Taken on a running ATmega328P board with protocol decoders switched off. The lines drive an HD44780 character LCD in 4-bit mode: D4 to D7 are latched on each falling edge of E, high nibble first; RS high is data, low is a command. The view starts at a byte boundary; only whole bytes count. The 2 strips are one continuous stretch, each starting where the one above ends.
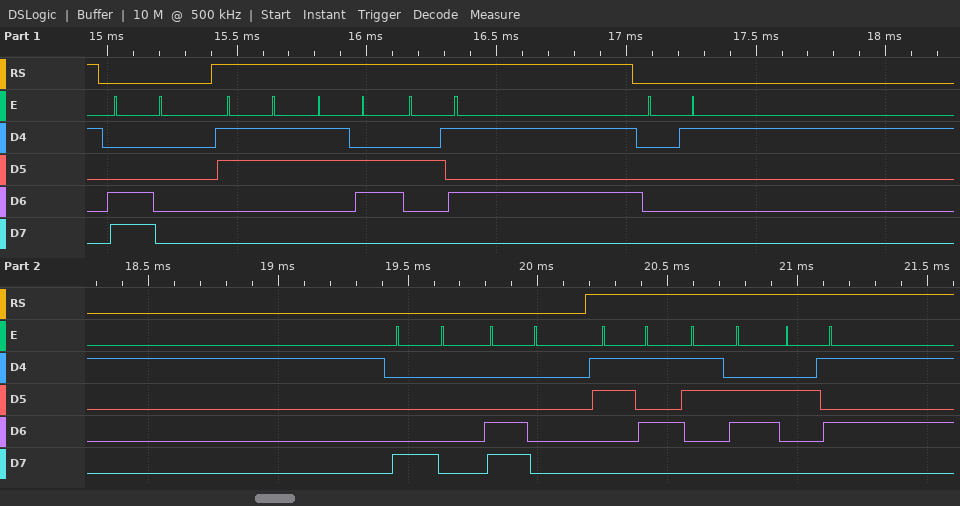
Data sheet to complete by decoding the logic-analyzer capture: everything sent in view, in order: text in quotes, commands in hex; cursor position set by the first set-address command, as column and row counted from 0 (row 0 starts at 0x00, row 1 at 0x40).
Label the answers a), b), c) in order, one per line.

a) 0xC0 "36%" 0x01 0x80 0xC0 "56%"
b) column 0, row 1
